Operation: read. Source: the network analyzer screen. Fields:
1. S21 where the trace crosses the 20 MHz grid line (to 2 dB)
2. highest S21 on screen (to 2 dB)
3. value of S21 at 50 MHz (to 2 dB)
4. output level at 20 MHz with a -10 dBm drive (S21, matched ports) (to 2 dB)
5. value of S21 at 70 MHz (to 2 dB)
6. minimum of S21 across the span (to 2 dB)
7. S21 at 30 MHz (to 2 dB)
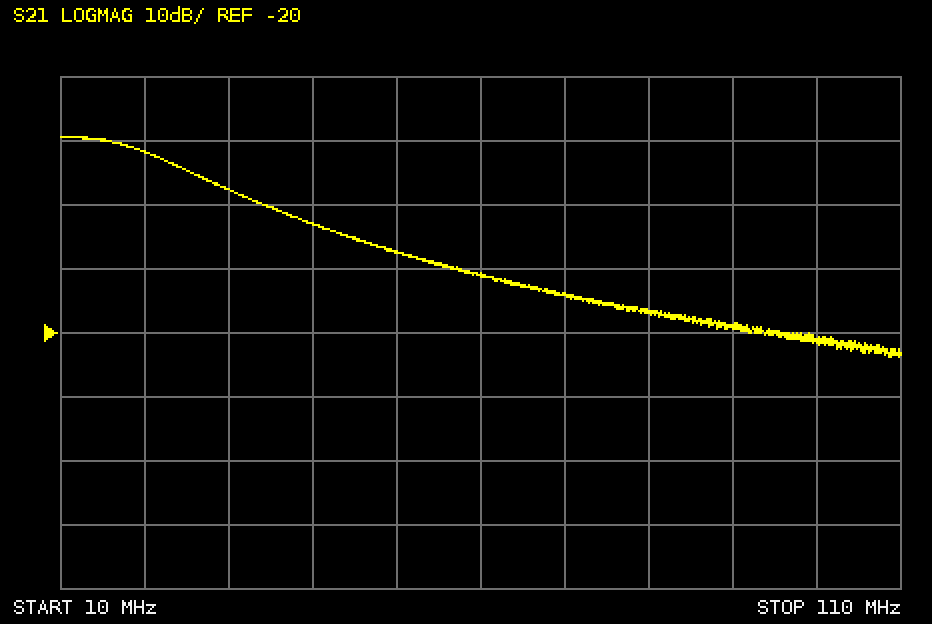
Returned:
8 dB
10 dB
-8 dB
-2 dBm
-14 dB
-24 dB
2 dB
